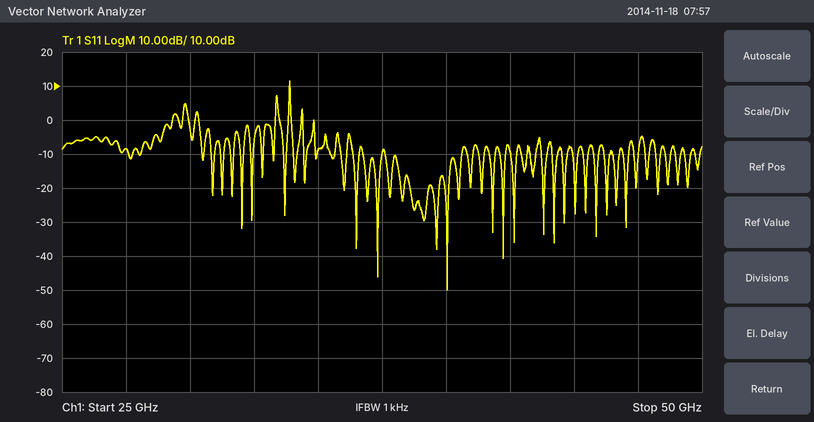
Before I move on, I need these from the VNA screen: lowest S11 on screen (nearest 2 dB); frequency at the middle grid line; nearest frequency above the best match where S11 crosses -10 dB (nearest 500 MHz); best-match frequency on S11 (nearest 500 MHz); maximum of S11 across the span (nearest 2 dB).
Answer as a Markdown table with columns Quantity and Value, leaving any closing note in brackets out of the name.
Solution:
| Quantity | Value |
|---|---|
| lowest S11 on screen | -50 dB |
| frequency at the middle grid line | 37.5 GHz |
| nearest frequency above the best match where S11 crosses -10 dB | 40.5 GHz |
| best-match frequency on S11 | 40.0 GHz |
| maximum of S11 across the span | 12 dB |
